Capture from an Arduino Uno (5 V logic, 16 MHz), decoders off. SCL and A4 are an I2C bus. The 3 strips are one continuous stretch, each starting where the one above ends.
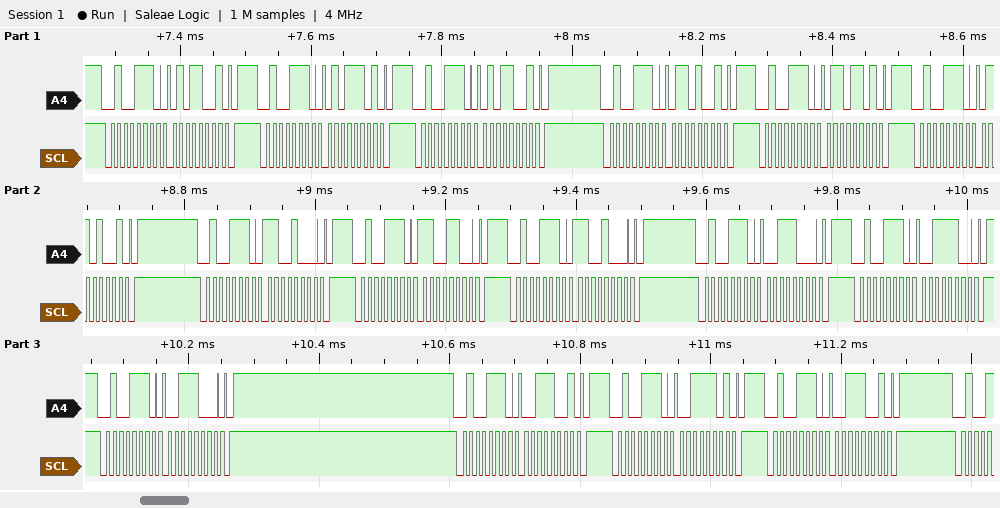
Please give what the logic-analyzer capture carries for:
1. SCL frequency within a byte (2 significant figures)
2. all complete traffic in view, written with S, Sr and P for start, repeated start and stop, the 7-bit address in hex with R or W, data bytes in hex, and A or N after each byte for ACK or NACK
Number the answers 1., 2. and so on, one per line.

1. 100 kHz
2. S 27W A 59 A P S 27W A 5D A P S 27W A 59 A P S 27W A 69 A P S 27W A 6D A P S 27W A 69 A P S 27W A C8 A P S 27W A CC A P S 27W A C8 A P S 27W A 38 A P S 27W A 3C A P S 27W A 38 A P S 27W A 39 A P S 27W A 3D A P S 27W A 39 A P
